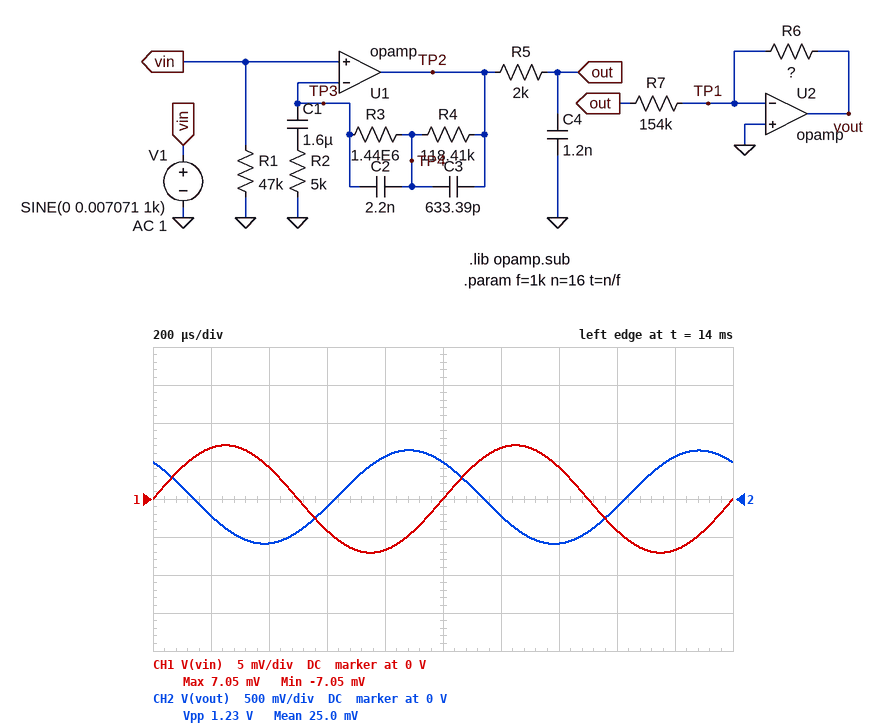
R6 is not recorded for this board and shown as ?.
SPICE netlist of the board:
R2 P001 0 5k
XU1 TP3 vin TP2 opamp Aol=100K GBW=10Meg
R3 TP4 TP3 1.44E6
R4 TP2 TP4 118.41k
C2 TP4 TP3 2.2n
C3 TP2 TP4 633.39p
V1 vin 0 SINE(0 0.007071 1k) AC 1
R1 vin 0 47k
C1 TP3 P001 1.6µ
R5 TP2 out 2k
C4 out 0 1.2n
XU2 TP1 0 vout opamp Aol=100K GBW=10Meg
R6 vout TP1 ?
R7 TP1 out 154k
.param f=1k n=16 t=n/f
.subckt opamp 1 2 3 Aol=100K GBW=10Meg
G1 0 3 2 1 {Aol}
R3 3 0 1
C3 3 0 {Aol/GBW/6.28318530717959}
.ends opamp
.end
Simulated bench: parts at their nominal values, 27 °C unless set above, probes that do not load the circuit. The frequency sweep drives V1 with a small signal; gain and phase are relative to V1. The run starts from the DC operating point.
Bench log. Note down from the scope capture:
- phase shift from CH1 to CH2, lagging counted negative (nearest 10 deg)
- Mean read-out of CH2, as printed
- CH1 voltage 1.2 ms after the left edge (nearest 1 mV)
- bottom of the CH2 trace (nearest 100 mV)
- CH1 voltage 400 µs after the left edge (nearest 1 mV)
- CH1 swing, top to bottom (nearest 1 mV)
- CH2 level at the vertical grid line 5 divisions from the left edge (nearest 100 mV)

130 deg
25.0 mV
7 mV
-600 mV
4 mV
14 mV
500 mV
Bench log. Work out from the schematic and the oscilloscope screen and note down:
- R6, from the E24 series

430 kΩ
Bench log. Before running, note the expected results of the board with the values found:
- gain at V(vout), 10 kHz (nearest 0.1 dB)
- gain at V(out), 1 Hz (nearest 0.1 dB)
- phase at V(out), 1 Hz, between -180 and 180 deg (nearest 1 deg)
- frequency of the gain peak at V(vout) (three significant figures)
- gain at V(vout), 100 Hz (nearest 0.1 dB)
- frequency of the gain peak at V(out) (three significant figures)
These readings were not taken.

25.0 dB
23.8 dB
82 deg
31.7 Hz
51.7 dB
31.7 Hz
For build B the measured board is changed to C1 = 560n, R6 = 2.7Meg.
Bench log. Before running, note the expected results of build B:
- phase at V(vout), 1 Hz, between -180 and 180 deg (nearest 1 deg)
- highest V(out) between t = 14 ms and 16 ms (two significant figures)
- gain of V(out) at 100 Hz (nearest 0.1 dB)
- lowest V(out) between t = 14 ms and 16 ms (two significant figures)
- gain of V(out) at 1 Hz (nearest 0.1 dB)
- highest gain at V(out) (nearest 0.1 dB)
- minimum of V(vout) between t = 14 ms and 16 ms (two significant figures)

-102 deg
220 mV
41.8 dB
-220 mV
14.9 dB
43.3 dB
-3.8 V
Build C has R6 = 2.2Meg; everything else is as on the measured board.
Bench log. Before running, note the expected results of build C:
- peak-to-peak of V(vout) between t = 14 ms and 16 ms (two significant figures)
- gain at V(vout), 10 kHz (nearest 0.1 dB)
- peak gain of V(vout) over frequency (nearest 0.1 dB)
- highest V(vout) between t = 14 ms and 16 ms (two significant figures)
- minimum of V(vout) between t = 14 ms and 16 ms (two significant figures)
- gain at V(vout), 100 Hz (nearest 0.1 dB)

6.3 V
39.2 dB
70.0 dB
3.3 V
-3.0 V
65.9 dB
